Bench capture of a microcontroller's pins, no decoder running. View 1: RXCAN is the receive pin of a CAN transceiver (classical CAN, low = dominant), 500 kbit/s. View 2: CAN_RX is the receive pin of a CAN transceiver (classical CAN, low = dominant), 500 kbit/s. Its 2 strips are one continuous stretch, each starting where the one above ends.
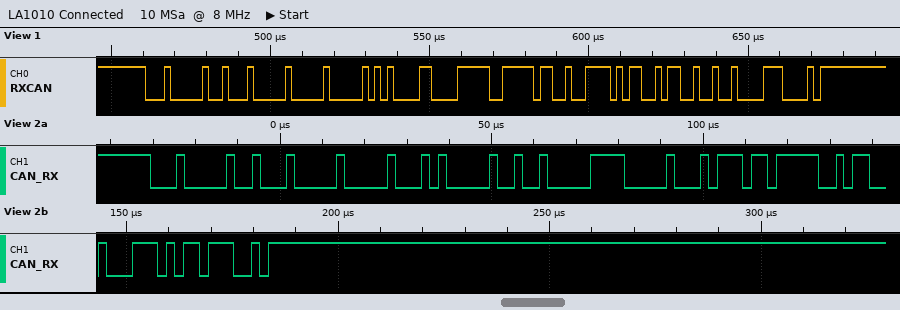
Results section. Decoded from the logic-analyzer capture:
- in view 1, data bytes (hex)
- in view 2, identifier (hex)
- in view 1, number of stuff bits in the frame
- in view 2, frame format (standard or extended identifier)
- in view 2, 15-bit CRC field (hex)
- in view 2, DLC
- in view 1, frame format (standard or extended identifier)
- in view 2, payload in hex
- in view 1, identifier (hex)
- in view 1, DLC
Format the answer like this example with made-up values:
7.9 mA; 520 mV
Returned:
00 05 0C 3E FE 4F 59 64; 0x101; 6; standard; 0x3ADC; 8; standard; 00 28 09 07 00 BB 7D 64; 0x101; 8
